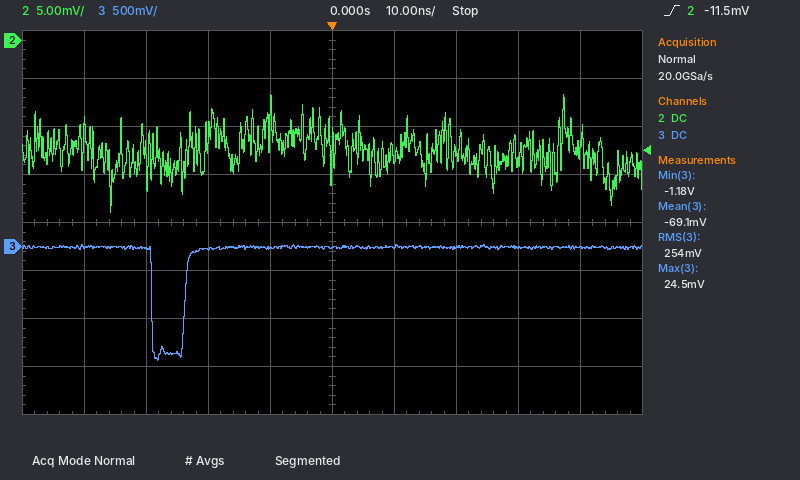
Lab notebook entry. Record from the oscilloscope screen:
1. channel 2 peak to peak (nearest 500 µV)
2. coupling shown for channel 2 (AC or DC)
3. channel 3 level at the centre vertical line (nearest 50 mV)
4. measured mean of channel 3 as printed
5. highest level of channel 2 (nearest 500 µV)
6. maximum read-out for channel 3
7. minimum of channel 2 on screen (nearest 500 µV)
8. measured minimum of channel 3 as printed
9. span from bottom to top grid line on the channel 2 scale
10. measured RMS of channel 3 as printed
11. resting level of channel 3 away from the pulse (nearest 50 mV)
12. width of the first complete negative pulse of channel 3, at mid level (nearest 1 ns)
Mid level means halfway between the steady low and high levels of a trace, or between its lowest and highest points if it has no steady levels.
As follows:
12.5 mV
DC
0 mV
-69.1 mV
-5.5 mV
24.5 mV
-18.0 mV
-1.18 V
40 mV
254 mV
0 mV
5 ns
